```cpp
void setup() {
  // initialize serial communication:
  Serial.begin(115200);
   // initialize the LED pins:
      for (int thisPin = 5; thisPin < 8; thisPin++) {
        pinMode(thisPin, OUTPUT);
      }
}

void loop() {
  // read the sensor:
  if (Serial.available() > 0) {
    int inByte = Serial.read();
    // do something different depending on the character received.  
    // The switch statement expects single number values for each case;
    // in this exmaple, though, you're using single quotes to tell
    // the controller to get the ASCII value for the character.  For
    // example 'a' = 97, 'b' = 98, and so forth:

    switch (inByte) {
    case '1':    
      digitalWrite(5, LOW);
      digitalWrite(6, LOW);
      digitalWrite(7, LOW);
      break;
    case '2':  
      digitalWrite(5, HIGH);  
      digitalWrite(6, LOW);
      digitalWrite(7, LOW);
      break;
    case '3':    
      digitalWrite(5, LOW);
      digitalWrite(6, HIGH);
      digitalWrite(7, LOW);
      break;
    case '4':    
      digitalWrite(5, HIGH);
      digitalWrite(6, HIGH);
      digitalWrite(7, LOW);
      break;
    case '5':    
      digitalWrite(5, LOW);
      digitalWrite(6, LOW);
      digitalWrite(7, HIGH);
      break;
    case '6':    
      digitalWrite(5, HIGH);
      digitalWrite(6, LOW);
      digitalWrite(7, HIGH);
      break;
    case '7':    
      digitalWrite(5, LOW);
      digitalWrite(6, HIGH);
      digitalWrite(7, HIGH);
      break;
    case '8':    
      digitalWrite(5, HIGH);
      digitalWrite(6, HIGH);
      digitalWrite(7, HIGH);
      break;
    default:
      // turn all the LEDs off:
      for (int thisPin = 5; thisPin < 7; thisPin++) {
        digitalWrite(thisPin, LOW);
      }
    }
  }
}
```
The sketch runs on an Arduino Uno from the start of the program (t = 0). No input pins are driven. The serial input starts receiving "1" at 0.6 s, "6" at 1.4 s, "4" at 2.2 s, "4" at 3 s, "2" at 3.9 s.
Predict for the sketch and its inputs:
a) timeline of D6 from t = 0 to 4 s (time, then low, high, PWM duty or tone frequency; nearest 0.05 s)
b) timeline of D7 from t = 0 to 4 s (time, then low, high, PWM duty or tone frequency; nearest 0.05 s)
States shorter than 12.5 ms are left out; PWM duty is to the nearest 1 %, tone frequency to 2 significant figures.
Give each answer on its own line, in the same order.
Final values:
0 s low; 2.2 s high; 3.9 s low
0 s low; 1.4 s high; 2.2 s low
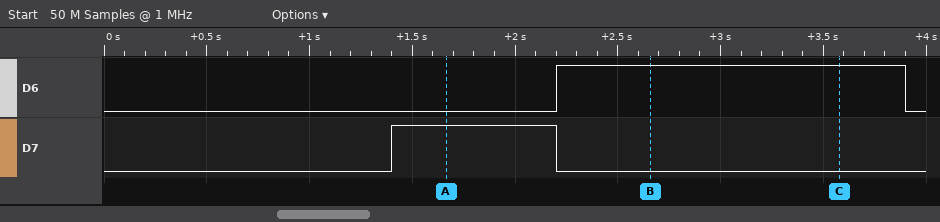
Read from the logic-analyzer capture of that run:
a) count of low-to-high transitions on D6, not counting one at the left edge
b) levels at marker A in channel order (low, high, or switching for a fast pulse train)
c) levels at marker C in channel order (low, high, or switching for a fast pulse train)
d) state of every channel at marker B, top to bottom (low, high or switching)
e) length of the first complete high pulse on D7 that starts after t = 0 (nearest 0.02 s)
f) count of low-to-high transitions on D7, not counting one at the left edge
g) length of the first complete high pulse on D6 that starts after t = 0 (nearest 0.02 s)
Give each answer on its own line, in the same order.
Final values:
1
D6 low, D7 high
D6 high, D7 low
D6 high, D7 low
0.80 s
1
1.70 s
